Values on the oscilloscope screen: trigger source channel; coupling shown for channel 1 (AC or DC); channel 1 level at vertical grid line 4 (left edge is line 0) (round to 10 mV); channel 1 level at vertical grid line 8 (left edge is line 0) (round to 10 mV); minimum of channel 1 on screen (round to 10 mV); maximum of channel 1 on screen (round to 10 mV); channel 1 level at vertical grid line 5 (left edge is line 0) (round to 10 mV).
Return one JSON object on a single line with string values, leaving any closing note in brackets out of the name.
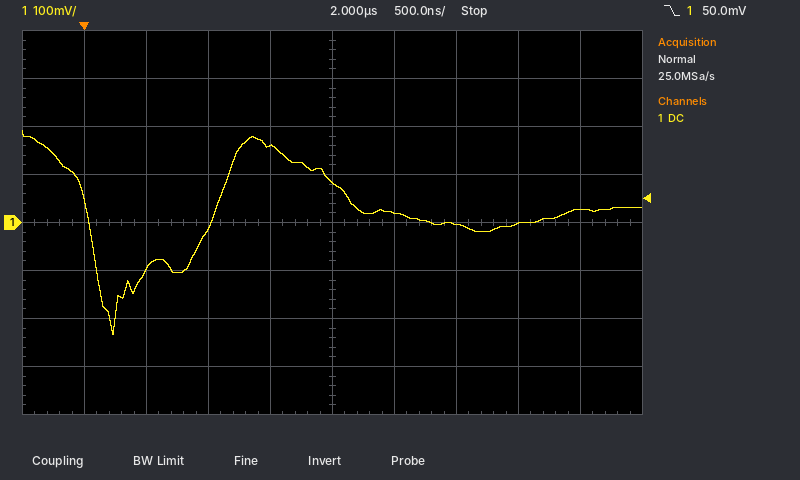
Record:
{"trigger source channel": "channel 1", "coupling shown for channel 1": "DC", "channel 1 level at vertical grid line 4 (left edge is line 0)": "160 mV", "channel 1 level at vertical grid line 8 (left edge is line 0)": "0 mV", "minimum of channel 1 on screen": "-230 mV", "maximum of channel 1 on screen": "190 mV", "channel 1 level at vertical grid line 5 (left edge is line 0)": "80 mV"}
